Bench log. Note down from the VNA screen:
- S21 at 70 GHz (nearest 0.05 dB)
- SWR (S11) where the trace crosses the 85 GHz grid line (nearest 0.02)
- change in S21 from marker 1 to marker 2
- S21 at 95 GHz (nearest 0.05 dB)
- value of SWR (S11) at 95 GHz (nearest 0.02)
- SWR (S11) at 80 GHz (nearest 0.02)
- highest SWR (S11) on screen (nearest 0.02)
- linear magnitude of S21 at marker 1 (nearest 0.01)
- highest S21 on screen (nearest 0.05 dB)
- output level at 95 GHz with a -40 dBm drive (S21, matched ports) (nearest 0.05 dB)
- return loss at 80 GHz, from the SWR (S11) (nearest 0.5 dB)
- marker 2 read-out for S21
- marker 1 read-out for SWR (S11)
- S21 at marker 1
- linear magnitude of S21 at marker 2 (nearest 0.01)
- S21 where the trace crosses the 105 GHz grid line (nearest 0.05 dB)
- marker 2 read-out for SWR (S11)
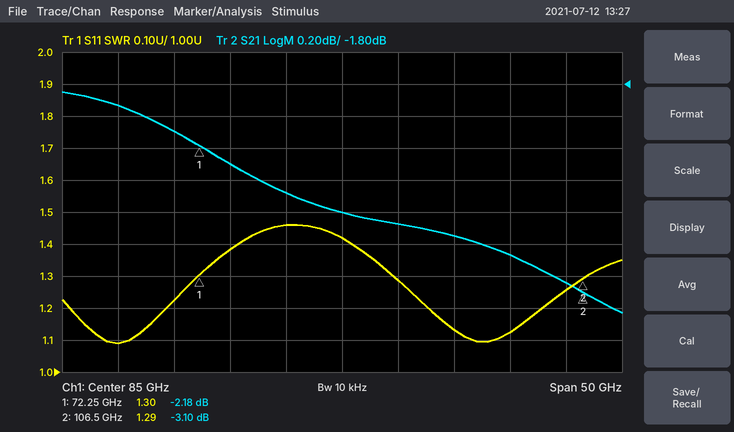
-2.10 dB
1.42
-0.92 dB
-2.75 dB
1.14
1.46
1.46
0.78
-1.85 dB
-42.75 dBm
14.5 dB
-3.10 dB
1.30
-2.18 dB
0.70
-3.05 dB
1.29
